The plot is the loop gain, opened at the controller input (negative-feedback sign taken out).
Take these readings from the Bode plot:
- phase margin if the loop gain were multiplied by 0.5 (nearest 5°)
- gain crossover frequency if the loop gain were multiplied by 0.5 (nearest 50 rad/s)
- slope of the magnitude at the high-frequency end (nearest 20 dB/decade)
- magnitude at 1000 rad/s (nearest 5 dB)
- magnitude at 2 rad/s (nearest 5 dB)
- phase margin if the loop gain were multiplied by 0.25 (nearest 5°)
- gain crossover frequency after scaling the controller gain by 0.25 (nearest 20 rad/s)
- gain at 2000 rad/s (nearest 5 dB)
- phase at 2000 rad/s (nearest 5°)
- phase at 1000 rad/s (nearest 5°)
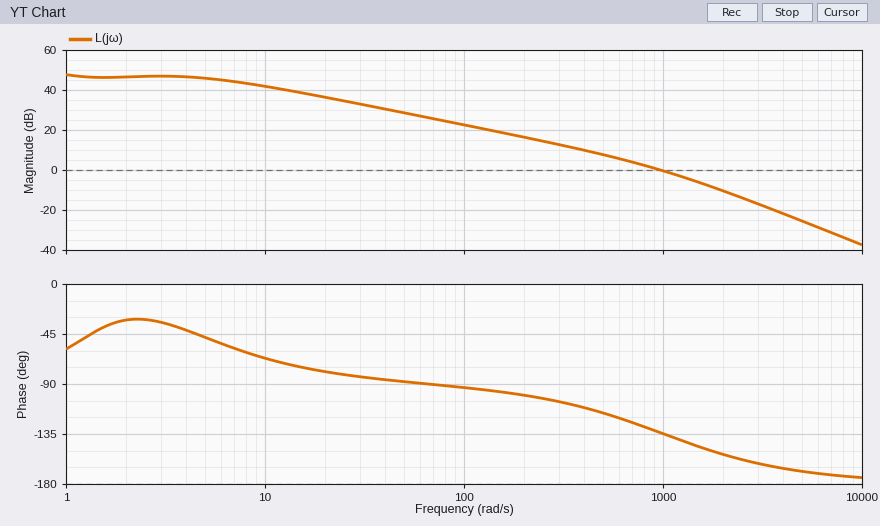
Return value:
60°
600 rad/s
-40 dB/decade
0 dB
45 dB
75°
320 rad/s
-10 dB
-155°
-135°
